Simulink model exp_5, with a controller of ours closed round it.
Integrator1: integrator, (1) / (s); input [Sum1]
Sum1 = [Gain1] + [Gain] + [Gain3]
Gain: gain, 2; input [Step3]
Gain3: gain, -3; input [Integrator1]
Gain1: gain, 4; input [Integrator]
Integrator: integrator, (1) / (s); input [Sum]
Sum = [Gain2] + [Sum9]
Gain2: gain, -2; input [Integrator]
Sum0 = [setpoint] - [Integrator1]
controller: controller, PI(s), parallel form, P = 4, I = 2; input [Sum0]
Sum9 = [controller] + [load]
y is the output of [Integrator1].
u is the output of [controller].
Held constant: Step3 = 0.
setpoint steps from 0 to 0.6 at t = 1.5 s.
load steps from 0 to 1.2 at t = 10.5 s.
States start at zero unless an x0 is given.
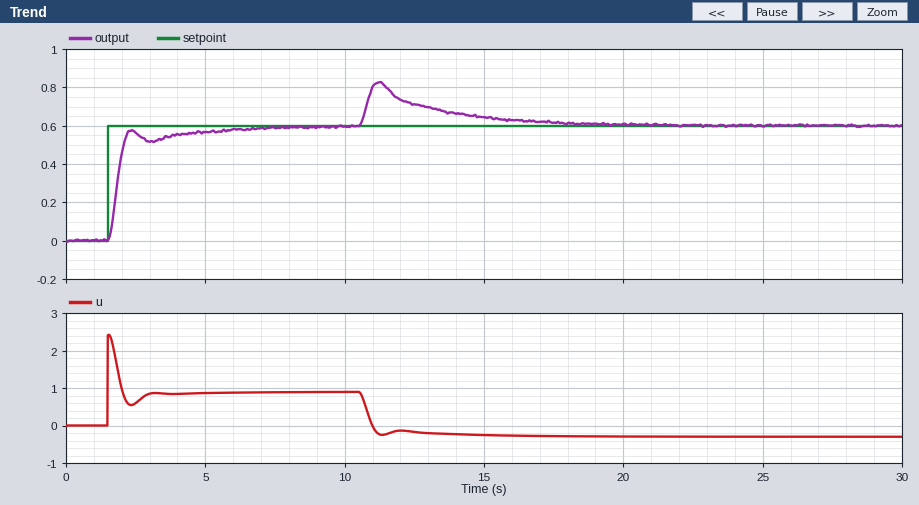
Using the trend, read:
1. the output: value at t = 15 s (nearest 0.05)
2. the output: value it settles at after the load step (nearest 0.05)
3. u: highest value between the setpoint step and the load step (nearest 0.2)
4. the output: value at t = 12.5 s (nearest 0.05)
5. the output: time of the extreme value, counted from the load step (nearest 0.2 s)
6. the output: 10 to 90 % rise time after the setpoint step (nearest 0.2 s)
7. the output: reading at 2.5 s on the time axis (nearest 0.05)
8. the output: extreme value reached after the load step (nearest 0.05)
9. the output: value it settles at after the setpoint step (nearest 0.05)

0.65
0.60
2.4
0.70
0.8 s
0.6 s
0.55
0.85
0.60
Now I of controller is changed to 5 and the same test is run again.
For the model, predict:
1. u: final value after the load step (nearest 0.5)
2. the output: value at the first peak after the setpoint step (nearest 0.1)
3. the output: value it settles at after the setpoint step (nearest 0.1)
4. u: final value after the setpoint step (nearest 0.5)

-0.5
0.7
0.6
1.0
